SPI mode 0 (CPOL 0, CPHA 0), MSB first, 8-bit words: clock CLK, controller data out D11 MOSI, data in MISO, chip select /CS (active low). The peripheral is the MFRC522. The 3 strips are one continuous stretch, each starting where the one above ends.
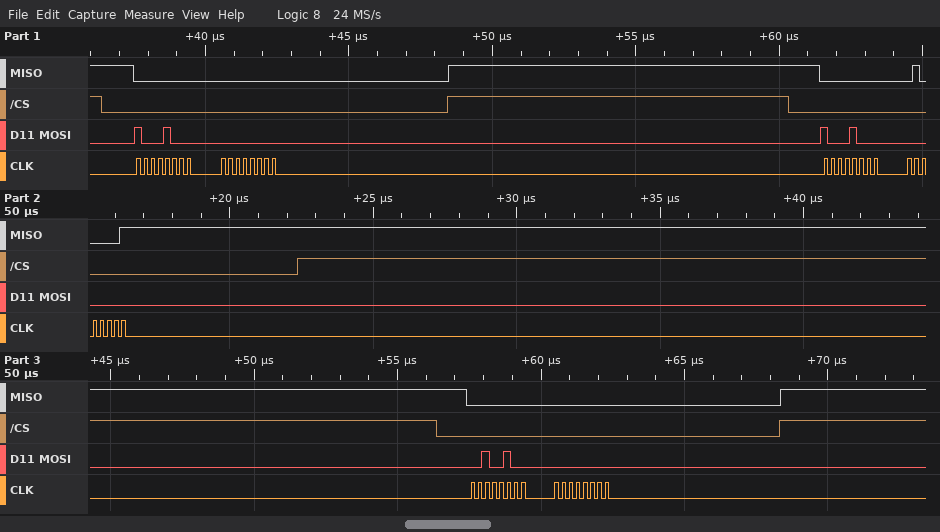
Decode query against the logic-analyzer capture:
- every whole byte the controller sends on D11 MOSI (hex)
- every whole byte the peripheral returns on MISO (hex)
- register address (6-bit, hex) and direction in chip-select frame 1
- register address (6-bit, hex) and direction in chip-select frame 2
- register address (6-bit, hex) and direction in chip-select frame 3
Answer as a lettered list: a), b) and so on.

a) 88 00 88 00 24 00
b) 00 00 00 41 00 00
c) 0x04 read
d) 0x04 read
e) 0x12 write
